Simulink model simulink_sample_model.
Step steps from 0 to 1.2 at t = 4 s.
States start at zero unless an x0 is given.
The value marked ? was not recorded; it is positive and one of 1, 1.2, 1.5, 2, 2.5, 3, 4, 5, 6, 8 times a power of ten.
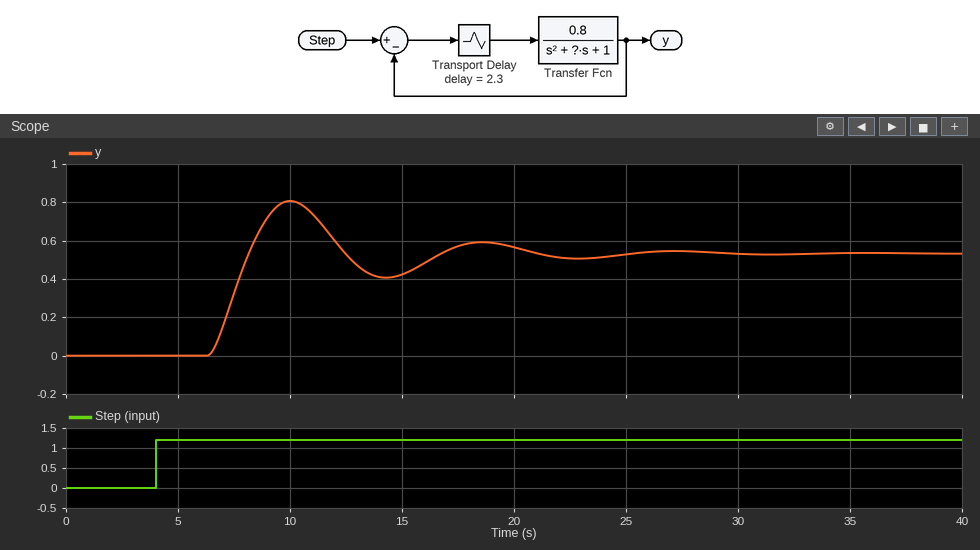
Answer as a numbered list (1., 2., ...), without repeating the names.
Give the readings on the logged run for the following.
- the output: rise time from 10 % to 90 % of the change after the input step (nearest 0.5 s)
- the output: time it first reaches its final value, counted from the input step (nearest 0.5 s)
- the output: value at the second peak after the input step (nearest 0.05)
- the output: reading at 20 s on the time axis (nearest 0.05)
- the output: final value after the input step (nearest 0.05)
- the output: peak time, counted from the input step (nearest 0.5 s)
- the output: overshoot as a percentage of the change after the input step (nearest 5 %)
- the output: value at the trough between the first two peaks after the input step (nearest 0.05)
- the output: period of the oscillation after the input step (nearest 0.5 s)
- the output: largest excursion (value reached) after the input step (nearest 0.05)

1. 1.5 s
2. 4.0 s
3. 0.60
4. 0.55
5. 0.55
6. 6.0 s
7. 50 %
8. 0.40
9. 8.5 s
10. 0.80
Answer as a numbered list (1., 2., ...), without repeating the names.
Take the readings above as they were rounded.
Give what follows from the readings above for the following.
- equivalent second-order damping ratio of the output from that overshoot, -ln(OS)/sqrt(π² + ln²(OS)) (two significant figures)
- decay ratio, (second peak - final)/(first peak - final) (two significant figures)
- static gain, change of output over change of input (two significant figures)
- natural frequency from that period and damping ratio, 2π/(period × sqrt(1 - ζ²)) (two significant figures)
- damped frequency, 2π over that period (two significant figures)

1. 0.22
2. 0.20
3. 0.46
4. 0.76 rad/s
5. 0.74 rad/s
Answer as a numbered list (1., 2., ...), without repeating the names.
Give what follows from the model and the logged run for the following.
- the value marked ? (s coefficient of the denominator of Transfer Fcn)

1. 2
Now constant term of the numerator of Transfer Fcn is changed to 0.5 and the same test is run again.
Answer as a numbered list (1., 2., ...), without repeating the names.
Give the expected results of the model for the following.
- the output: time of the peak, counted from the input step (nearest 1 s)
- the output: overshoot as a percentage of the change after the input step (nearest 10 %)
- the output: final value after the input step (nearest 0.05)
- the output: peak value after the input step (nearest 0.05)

1. 6 s
2. 30 %
3. 0.40
4. 0.50
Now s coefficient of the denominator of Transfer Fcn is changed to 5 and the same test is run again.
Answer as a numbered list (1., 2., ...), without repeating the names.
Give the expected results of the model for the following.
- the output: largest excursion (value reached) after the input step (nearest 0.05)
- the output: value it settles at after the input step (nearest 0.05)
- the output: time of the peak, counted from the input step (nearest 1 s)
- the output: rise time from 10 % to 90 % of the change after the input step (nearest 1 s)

1. 0.55
2. 0.55
3. 9 s
4. 3 s
